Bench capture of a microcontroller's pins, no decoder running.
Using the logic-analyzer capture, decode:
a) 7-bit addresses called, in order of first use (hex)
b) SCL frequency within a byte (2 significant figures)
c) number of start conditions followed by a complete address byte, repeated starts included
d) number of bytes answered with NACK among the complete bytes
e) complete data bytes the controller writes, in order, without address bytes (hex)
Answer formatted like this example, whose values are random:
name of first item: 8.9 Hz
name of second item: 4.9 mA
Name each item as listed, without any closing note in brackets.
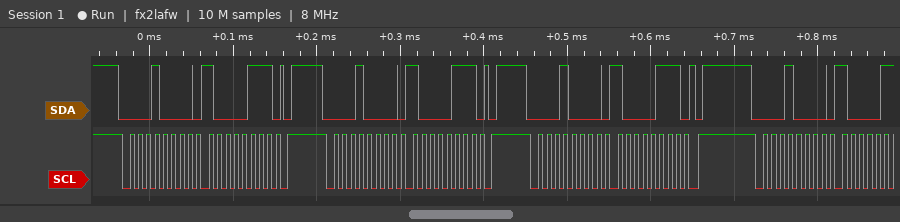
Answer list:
7-bit addresses called, in order of first use: 0x08
SCL frequency within a byte: 100 kHz
number of start conditions followed by a complete address byte, repeated starts included: 4
number of bytes answered with NACK among the complete bytes: 0
complete data bytes the controller writes, in order, without address bytes: 87 87 87
